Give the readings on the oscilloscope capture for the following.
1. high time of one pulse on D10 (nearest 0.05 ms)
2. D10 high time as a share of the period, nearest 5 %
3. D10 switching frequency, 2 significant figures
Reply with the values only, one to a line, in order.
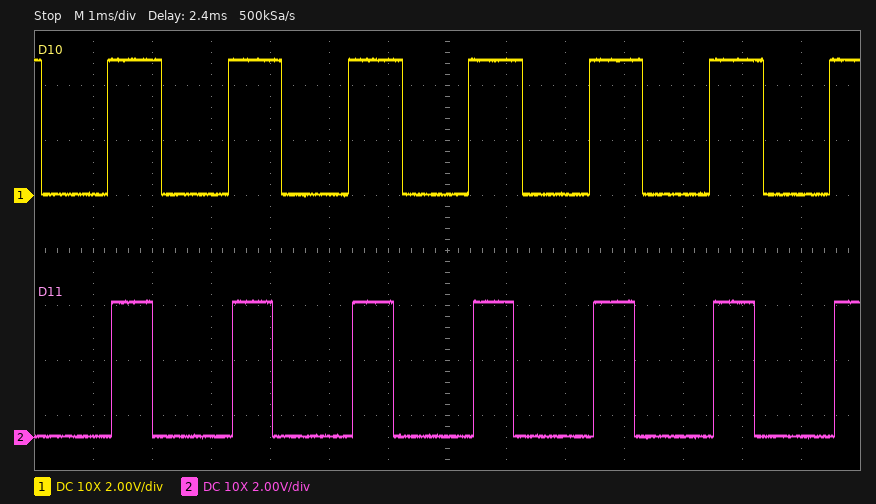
0.90 ms
45 %
490 Hz
